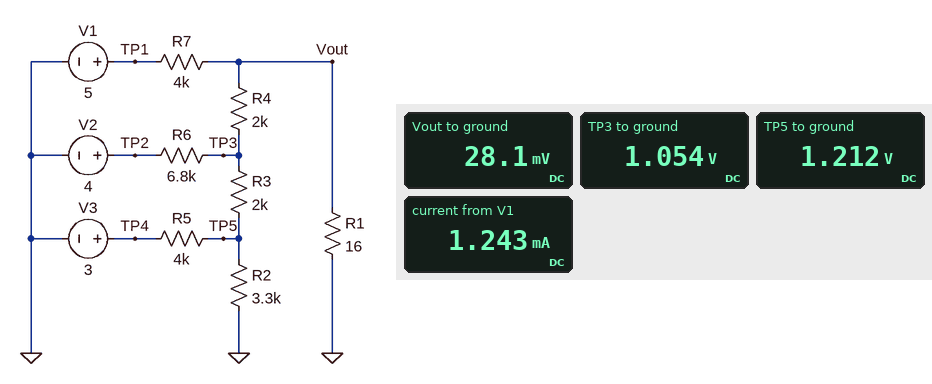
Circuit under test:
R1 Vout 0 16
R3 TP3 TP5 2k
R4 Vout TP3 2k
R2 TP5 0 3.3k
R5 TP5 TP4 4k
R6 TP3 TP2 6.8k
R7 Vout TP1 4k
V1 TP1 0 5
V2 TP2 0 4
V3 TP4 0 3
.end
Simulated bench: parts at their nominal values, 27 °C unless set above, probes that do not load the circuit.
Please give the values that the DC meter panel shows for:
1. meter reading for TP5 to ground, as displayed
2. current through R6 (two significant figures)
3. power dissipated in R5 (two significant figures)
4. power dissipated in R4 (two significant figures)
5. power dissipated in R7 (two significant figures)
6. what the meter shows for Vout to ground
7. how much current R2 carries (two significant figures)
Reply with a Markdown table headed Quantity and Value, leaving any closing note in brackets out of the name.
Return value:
| Quantity | Value |
|---|---|
| meter reading for TP5 to ground, as displayed | 1.212 V |
| current through R6 | 430 µA |
| power dissipated in R5 | 800 µW |
| power dissipated in R4 | 530 µW |
| power dissipated in R7 | 6.2 mW |
| what the meter shows for Vout to ground | 28.1 mV |
| how much current R2 carries | 370 µA |
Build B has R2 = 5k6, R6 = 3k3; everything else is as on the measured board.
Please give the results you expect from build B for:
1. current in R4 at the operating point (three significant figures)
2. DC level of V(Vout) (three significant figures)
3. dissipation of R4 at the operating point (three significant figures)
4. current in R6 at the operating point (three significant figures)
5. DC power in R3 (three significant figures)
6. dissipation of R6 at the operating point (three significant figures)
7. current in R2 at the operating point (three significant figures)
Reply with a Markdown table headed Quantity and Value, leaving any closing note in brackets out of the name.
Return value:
| Quantity | Value |
|---|---|
| current in R4 at the operating point | 773 µA |
| DC level of V(Vout) | 32.2 mV |
| dissipation of R4 at the operating point | 1.20 mW |
| current in R6 at the operating point | 734 µA |
| DC power in R3 | 3.12 µW |
| dissipation of R6 at the operating point | 1.78 mW |
| current in R2 at the operating point | 296 µA |
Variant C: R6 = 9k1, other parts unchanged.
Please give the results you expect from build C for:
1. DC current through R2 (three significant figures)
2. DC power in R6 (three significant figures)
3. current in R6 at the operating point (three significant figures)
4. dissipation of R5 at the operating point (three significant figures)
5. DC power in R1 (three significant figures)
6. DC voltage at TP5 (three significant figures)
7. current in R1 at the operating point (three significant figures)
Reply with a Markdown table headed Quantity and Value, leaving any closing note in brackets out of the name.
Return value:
| Quantity | Value |
|---|---|
| DC current through R2 | 349 µA |
| DC power in R6 | 1.04 mW |
| current in R6 at the operating point | 338 µA |
| dissipation of R5 at the operating point | 853 µW |
| DC power in R1 | 45.9 µW |
| DC voltage at TP5 | 1.15 V |
| current in R1 at the operating point | 1.69 mA |
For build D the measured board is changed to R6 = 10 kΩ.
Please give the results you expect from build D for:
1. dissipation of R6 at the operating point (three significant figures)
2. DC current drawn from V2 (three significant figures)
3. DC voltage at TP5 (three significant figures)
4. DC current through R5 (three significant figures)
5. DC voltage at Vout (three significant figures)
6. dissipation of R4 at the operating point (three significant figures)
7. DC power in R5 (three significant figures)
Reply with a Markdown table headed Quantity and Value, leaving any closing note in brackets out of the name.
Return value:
| Quantity | Value |
|---|---|
| dissipation of R6 at the operating point | 966 µW |
| DC current drawn from V2 | 311 µA |
| DC voltage at TP5 | 1.14 V |
| DC current through R5 | 466 µA |
| DC voltage at Vout | 26.8 mV |
| dissipation of R4 at the operating point | 374 µW |
| DC power in R5 | 869 µW |
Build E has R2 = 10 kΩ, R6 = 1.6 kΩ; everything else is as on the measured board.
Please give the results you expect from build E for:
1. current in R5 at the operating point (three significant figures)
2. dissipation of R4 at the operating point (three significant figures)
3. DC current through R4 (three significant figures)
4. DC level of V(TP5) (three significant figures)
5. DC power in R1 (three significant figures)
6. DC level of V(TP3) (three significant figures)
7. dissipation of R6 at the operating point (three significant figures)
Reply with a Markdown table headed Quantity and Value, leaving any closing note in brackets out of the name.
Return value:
| Quantity | Value |
|---|---|
| current in R5 at the operating point | 202 µA |
| dissipation of R4 at the operating point | 2.39 mW |
| DC current through R4 | 1.09 mA |
| DC level of V(TP5) | 2.19 V |
| DC power in R1 | 87.2 µW |
| DC level of V(TP3) | 2.22 V |
| dissipation of R6 at the operating point | 1.97 mW |
